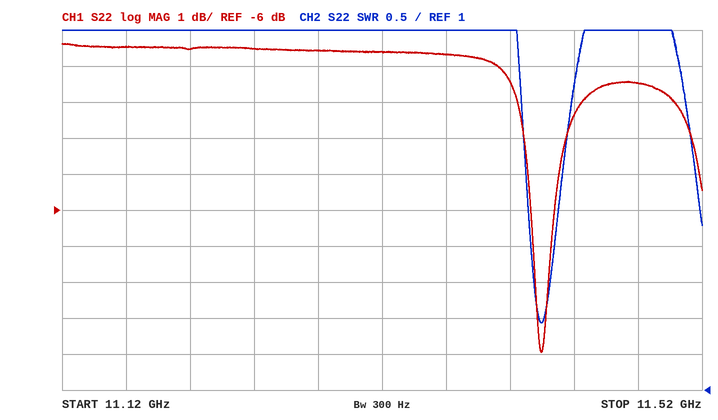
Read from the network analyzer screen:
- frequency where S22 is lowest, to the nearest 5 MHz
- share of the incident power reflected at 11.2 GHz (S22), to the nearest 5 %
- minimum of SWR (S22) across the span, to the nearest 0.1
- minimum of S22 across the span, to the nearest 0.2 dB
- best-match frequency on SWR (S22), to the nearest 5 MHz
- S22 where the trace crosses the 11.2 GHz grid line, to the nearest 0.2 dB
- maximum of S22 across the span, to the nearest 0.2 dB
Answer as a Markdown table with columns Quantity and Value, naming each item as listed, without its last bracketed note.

| Quantity | Value |
|---|---|
| frequency where S22 is lowest, to the nearest 5 MHz | 11.420 GHz |
| share of the incident power reflected at 11.2 GHz (S22), to the nearest 5 % | 70 % |
| minimum of SWR (S22) across the span, to the nearest 0.1 | 1.9 |
| minimum of S22 across the span, to the nearest 0.2 dB | -10.0 dB |
| best-match frequency on SWR (S22), to the nearest 5 MHz | 11.420 GHz |
| S22 where the trace crosses the 11.2 GHz grid line, to the nearest 0.2 dB | -1.6 dB |
| maximum of S22 across the span, to the nearest 0.2 dB | -1.4 dB |
